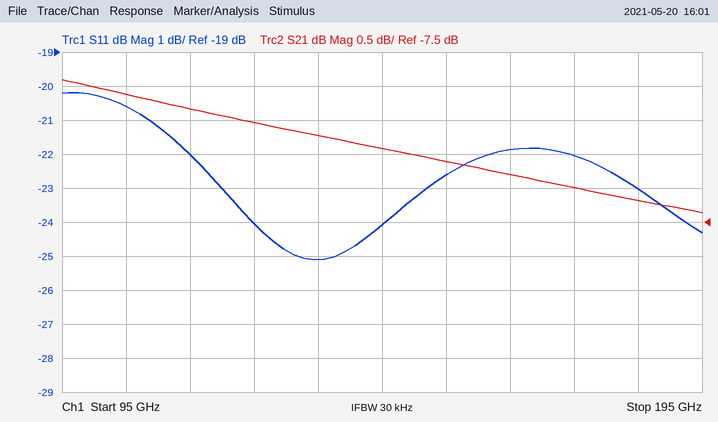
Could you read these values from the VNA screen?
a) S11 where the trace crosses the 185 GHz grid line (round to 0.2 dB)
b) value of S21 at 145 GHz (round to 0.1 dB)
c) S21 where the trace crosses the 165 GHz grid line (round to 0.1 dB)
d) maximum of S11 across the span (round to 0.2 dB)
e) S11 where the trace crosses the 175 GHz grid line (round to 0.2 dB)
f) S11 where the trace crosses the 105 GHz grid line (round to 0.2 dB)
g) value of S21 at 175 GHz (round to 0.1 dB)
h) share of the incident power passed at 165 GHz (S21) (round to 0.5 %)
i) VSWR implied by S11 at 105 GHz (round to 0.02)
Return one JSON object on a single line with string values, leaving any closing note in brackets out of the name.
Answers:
{"S11 where the trace crosses the 185 GHz grid line": "-23.0 dB", "value of S21 at 145 GHz": "-6.4 dB", "S21 where the trace crosses the 165 GHz grid line": "-6.8 dB", "maximum of S11 across the span": "-20.2 dB", "S11 where the trace crosses the 175 GHz grid line": "-22.0 dB", "S11 where the trace crosses the 105 GHz grid line": "-20.6 dB", "value of S21 at 175 GHz": "-7.0 dB", "share of the incident power passed at 165 GHz (S21)": "21.0 %", "VSWR implied by S11 at 105 GHz": "1.20"}
